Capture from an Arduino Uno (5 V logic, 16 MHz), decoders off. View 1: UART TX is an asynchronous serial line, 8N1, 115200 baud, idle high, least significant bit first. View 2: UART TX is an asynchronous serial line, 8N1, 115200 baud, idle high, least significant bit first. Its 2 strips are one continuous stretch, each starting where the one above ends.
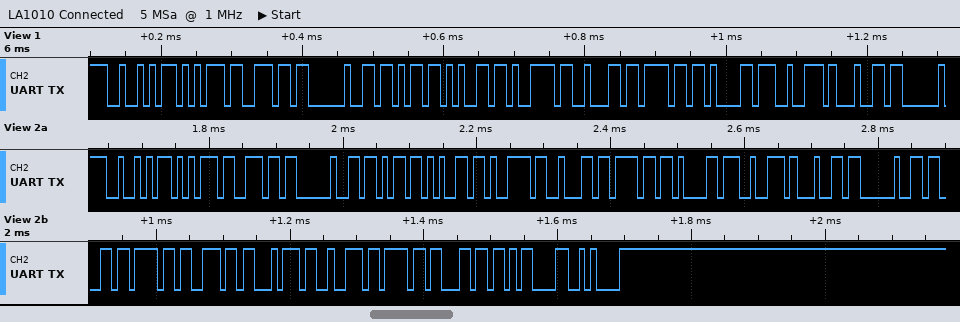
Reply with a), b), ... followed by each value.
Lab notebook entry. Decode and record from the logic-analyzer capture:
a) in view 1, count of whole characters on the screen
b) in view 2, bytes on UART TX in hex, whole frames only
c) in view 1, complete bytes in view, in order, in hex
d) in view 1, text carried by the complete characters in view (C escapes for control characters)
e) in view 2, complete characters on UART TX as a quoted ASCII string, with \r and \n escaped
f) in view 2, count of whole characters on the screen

a) 12
b) 52 75 6E 20 6B 65 79 62 6F 61 72 64 20 63 6F 6E 74 72 6F 6C 0D 0A
c) 52 75 6E 20 6B 65 79 62 6F 61 72 64
d) "Run keyboard"
e) "Run keyboard control\r\n"
f) 22
